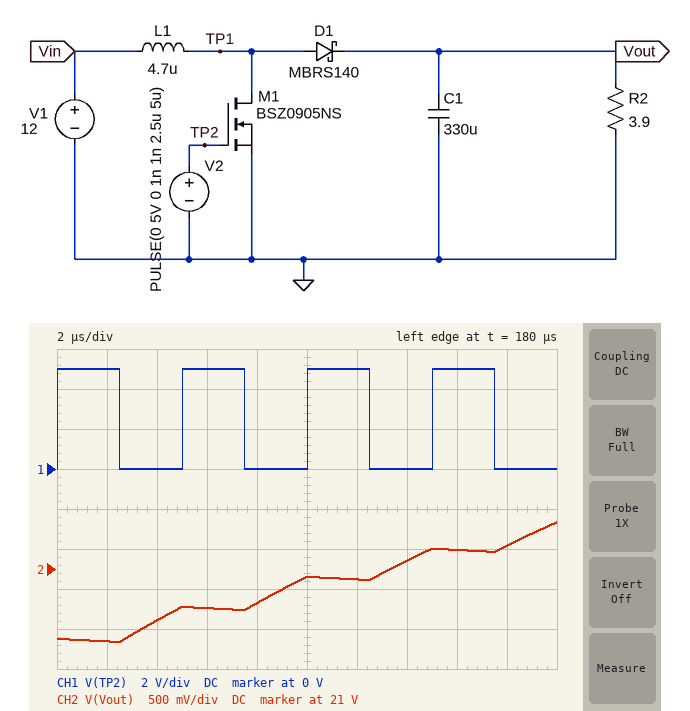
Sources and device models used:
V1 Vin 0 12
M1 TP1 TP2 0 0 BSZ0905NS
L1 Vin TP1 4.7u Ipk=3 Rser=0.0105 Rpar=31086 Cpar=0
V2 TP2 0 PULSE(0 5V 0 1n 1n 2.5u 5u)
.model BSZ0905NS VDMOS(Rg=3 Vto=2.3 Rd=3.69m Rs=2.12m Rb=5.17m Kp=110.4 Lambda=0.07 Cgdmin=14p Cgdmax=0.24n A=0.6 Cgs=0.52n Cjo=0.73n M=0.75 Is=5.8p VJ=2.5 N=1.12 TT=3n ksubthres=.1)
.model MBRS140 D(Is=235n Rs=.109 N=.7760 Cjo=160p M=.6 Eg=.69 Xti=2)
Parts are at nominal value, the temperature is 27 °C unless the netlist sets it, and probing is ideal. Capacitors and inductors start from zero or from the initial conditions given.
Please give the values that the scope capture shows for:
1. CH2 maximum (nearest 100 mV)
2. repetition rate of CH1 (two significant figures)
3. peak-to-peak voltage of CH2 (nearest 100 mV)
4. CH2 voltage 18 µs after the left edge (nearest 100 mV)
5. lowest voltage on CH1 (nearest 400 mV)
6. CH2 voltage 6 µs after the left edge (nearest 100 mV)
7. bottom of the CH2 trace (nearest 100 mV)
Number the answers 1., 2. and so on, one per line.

1. 21.6 V
2. 200 kHz
3. 1.5 V
4. 21.3 V
5. 0 V
6. 20.5 V
7. 20.1 V
